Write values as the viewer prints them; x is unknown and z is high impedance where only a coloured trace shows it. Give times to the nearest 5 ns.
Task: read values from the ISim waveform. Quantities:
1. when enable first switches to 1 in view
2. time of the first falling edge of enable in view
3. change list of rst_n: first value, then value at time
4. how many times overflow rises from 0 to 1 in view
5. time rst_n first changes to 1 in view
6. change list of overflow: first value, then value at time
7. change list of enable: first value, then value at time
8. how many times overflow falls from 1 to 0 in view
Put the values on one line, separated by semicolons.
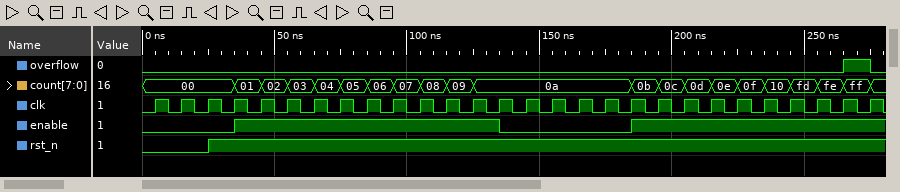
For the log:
35 ns; 135 ns; 0, 1 at 25 ns; 1; 25 ns; 0, 1 at 265 ns, 0 at 275 ns; 0, 1 at 35 ns, 0 at 135 ns, 1 at 185 ns; 1
